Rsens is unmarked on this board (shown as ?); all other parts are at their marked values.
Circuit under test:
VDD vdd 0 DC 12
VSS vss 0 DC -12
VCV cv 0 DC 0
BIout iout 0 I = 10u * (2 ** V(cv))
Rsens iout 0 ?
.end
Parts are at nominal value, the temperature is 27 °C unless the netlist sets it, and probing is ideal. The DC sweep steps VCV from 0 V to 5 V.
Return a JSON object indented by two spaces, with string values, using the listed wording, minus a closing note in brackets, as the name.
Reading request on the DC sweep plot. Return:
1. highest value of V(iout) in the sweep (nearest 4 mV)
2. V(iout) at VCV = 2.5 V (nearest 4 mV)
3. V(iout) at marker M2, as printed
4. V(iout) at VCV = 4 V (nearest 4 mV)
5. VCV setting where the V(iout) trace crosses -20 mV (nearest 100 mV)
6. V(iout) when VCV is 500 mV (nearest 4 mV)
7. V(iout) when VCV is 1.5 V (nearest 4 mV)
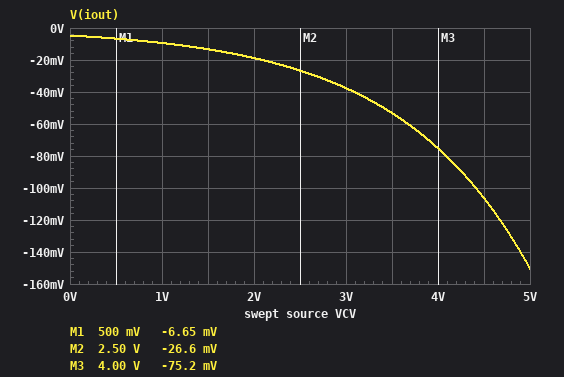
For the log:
{
  "highest value of V(iout) in the sweep": "-4 mV",
  "V(iout) at VCV = 2.5 V": "-28 mV",
  "V(iout) at marker M2, as printed": "-26.6 mV",
  "V(iout) at VCV = 4 V": "-76 mV",
  "VCV setting where the V(iout) trace crosses -20 mV": "2.1 V",
  "V(iout) when VCV is 500 mV": "-8 mV",
  "V(iout) when VCV is 1.5 V": "-12 mV"
}
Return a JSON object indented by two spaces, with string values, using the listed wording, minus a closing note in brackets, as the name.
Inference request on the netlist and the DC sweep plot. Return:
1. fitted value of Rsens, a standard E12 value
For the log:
{
  "fitted value of Rsens, a standard E12 value": "470 Ω"
}
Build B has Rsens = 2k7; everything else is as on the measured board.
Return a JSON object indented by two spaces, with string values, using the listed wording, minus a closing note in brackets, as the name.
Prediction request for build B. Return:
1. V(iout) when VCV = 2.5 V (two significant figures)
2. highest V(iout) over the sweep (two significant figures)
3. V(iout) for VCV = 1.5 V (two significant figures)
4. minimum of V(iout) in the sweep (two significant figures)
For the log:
{
  "V(iout) when VCV = 2.5 V": "-150 mV",
  "highest V(iout) over the sweep": "-27 mV",
  "V(iout) for VCV = 1.5 V": "-76 mV",
  "minimum of V(iout) in the sweep": "-860 mV"
}
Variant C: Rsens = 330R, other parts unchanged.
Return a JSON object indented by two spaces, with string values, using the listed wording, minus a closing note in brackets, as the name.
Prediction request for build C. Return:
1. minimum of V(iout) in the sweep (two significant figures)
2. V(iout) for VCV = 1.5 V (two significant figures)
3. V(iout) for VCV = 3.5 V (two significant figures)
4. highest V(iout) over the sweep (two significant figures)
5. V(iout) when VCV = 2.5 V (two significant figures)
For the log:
{
  "minimum of V(iout) in the sweep": "-110 mV",
  "V(iout) for VCV = 1.5 V": "-9.3 mV",
  "V(iout) for VCV = 3.5 V": "-37 mV",
  "highest V(iout) over the sweep": "-3.3 mV",
  "V(iout) when VCV = 2.5 V": "-19 mV"
}
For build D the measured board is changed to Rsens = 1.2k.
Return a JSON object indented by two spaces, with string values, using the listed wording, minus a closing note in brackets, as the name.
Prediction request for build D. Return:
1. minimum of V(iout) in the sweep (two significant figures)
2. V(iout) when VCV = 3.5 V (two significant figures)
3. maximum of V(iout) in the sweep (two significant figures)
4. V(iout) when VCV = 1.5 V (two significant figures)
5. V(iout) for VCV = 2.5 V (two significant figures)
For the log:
{
  "minimum of V(iout) in the sweep": "-380 mV",
  "V(iout) when VCV = 3.5 V": "-140 mV",
  "maximum of V(iout) in the sweep": "-12 mV",
  "V(iout) when VCV = 1.5 V": "-34 mV",
  "V(iout) for VCV = 2.5 V": "-68 mV"
}
